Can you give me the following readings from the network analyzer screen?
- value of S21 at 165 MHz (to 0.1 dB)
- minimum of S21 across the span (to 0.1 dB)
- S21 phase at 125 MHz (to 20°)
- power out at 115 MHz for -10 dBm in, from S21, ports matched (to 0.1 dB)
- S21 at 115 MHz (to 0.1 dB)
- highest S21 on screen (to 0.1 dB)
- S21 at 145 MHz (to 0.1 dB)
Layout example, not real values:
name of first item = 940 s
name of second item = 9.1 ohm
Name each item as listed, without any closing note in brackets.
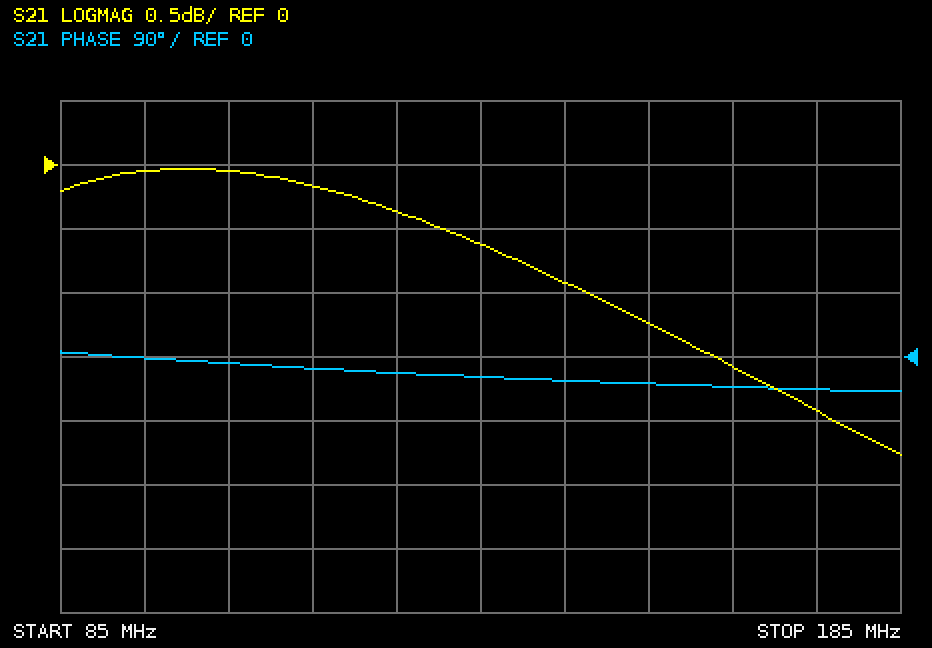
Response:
value of S21 at 165 MHz = -1.6 dB
minimum of S21 across the span = -2.3 dB
S21 phase at 125 MHz = -20°
power out at 115 MHz for -10 dBm in, from S21, ports matched = -10.2 dBm
S21 at 115 MHz = -0.2 dB
highest S21 on screen = 0.0 dB
S21 at 145 MHz = -0.9 dB
